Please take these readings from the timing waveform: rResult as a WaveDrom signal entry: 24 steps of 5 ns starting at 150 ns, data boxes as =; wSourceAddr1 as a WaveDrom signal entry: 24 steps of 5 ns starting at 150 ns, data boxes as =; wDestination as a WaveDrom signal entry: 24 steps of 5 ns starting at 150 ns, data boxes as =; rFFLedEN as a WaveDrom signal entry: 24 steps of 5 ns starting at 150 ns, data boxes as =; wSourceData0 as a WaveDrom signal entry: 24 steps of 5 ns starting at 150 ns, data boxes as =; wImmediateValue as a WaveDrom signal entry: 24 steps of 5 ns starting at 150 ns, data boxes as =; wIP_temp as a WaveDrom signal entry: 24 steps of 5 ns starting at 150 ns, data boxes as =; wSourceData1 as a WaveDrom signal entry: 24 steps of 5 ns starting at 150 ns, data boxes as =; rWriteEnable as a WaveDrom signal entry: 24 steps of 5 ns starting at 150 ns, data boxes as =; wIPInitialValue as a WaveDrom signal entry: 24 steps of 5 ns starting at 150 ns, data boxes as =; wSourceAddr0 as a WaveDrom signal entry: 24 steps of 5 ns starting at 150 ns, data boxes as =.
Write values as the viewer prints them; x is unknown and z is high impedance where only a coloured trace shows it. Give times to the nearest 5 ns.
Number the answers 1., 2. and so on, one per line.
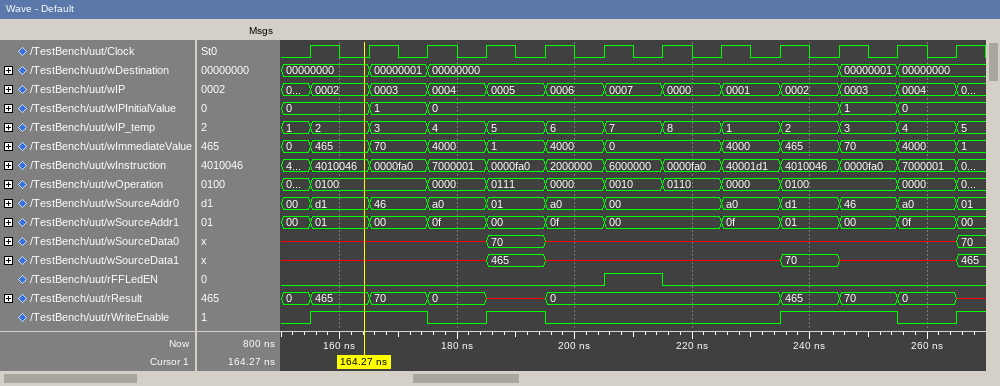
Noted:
1. {name: 'rResult', wave: '==.=.=.x.=.......=.=.=.x', data: '0 465 70 0 0 465 70 0'}
2. {name: 'wSourceAddr1', wave: '==.=.=.=.=.=...=.=.=.=.=', data: '00 01 00 0f 00 0f 00 0f 01 00 0f 00'}
3. {name: 'wDestination', wave: '=..=.=.............=.=..', data: '00000000 00000001 00000000 00000001 00000000'}
4. {name: 'rFFLedEN', wave: '0..........1.0..........'}
5. {name: 'wSourceData0', wave: 'x......=.x.............=', data: '70 70'}
6. {name: 'wImmediateValue', wave: '==.=.=.=.=.=...=.=.=.=.=', data: '0 465 70 4000 1 4000 0 4000 465 70 4000 1'}
7. {name: 'wIP_temp', wave: '==.=.=.=.=.=.=.=.=.=.=.=', data: '1 2 3 4 5 6 7 8 1 2 3 4 5'}
8. {name: 'wSourceData1', wave: 'x......=.x.......=.x...=', data: '465 70 465'}
9. {name: 'rWriteEnable', wave: '01...0.1.0.......1...0.1'}
10. {name: 'wIPInitialValue', wave: '=..=.=.............=.=..', data: '0 1 0 1 0'}
11. {name: 'wSourceAddr0', wave: '==.=.=.=.=.=...=.=.=.=.=', data: '00 d1 46 a0 01 a0 00 a0 d1 46 a0 01'}
